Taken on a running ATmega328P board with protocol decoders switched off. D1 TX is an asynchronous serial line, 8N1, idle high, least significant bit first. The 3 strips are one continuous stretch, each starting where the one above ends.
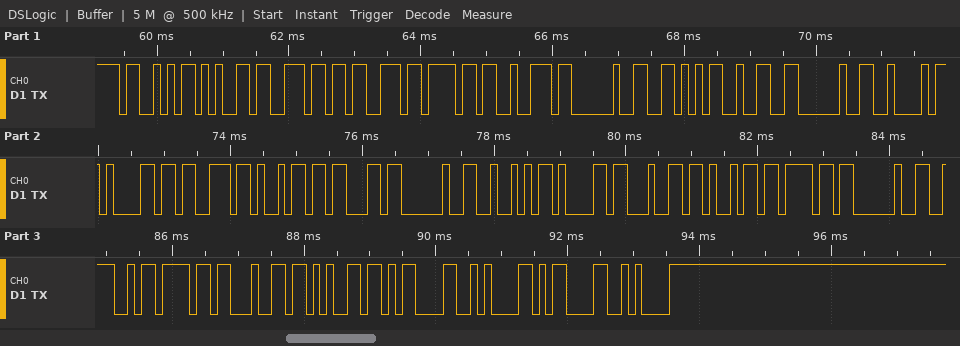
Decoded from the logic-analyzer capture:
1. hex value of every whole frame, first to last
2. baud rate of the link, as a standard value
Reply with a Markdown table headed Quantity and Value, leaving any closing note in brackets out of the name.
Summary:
| Quantity | Value |
|---|---|
| hex value of every whole frame, first to last | 0x53 0x65 0x6E 0x73 0x6F 0x72 0x20 0x56 0x32 0x20 0x42 0x61 0x73 0x69 0x63 0x20 0x52 0x61 0x64 0x69 0x6F 0x20 0x4E 0x6F 0x64 0x65 0x0D 0x0A 0x0D 0x0A |
| baud rate of the link, as a standard value | 9600 baud |
